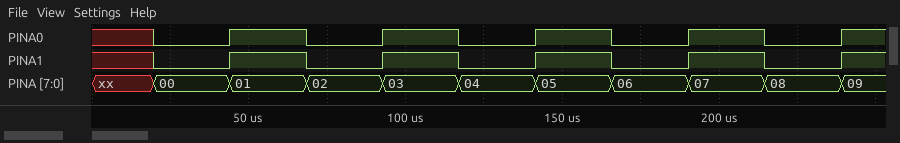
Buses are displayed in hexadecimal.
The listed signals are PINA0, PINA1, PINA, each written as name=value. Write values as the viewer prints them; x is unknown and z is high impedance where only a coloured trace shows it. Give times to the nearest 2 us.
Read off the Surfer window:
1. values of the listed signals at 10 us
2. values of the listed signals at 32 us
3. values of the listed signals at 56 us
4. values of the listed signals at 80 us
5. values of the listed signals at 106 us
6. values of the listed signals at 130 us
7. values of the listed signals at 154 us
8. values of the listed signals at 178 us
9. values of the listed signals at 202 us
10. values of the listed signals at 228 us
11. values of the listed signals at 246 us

PINA0=x, PINA1=x, PINA=xx
PINA0=0, PINA1=0, PINA=00
PINA0=1, PINA1=1, PINA=01
PINA0=0, PINA1=0, PINA=02
PINA0=1, PINA1=1, PINA=03
PINA0=0, PINA1=0, PINA=04
PINA0=1, PINA1=1, PINA=05
PINA0=0, PINA1=0, PINA=06
PINA0=1, PINA1=1, PINA=07
PINA0=0, PINA1=0, PINA=08
PINA0=1, PINA1=1, PINA=09
